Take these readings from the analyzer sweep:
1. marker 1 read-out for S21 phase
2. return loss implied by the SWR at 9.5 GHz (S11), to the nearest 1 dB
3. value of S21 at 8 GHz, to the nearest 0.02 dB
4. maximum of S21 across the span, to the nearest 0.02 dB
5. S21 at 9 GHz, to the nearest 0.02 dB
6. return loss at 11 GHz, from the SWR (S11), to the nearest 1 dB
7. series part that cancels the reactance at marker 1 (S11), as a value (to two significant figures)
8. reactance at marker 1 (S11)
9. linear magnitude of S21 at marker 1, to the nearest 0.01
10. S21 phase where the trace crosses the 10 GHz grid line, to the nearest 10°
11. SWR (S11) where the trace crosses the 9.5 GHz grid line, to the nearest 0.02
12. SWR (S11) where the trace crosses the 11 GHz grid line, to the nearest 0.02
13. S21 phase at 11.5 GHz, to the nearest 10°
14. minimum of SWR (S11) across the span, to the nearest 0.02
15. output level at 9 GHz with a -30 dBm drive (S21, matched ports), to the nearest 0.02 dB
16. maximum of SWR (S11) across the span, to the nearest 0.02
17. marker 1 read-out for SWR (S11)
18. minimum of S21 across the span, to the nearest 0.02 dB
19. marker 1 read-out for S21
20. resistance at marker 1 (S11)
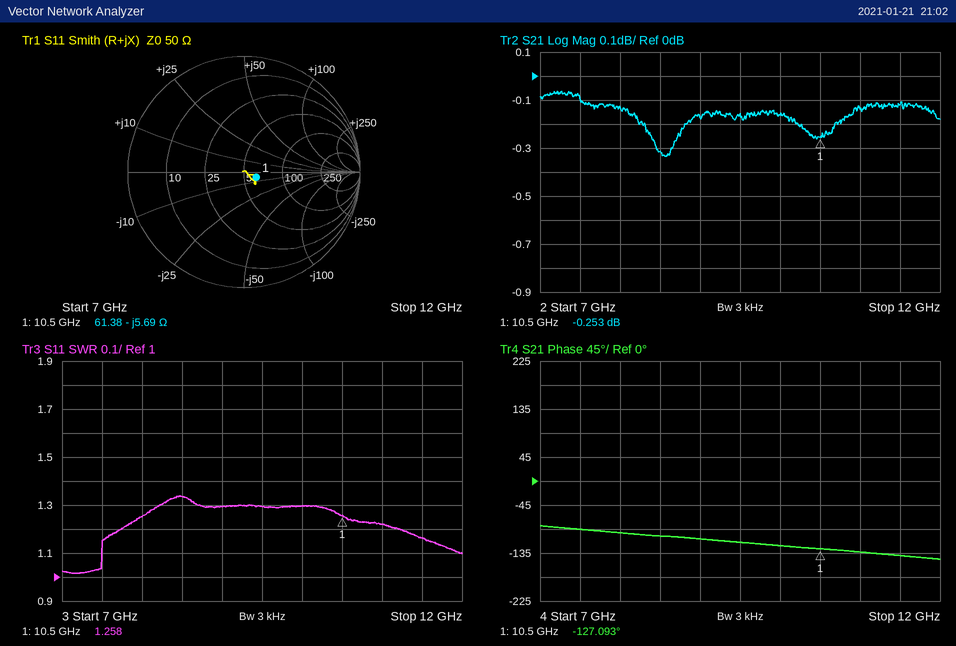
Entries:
-127.093°
18 dB
-0.14 dB
-0.06 dB
-0.18 dB
20 dB
86 pH
-5.69 Ω
0.97
-120°
1.30
1.22
-140°
1.02
-30.18 dBm
1.34
1.258
-0.34 dB
-0.253 dB
61.38 Ω
